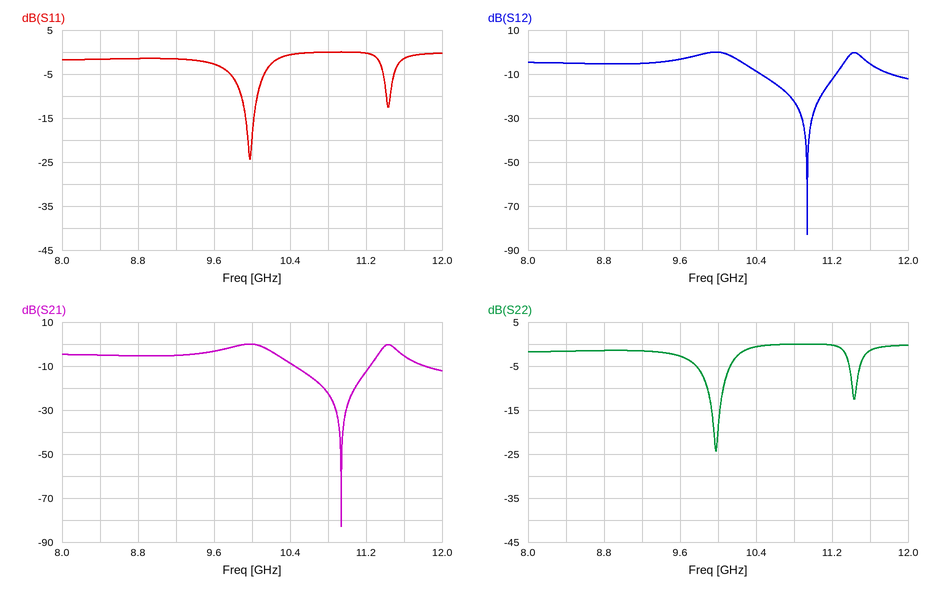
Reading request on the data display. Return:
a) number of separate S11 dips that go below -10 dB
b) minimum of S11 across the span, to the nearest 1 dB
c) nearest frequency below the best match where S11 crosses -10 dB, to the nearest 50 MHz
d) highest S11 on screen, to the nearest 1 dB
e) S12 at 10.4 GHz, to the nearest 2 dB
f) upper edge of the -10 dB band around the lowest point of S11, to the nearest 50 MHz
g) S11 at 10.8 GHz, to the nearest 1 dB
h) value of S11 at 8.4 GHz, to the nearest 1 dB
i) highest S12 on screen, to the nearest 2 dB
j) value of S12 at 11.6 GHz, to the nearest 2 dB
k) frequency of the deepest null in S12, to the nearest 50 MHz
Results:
2
-24 dB
9.90 GHz
0 dB
-8 dB
10.05 GHz
0 dB
-2 dB
0 dB
-6 dB
10.95 GHz
